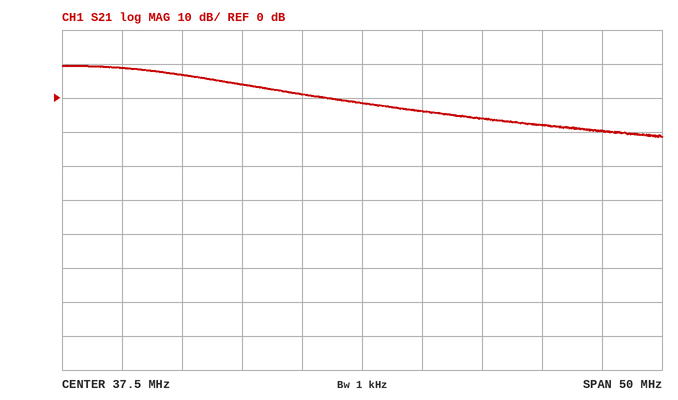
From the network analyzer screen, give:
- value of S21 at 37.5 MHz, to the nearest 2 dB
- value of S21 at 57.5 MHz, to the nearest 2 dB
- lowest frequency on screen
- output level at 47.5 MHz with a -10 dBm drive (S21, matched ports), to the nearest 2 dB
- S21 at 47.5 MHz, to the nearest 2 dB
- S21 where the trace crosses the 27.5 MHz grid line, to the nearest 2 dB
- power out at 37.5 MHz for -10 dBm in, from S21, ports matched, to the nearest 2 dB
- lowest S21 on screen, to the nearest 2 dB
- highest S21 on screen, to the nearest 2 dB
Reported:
-2 dB
-10 dB
12.5 MHz
-16 dBm
-6 dB
4 dB
-12 dBm
-12 dB
10 dB
